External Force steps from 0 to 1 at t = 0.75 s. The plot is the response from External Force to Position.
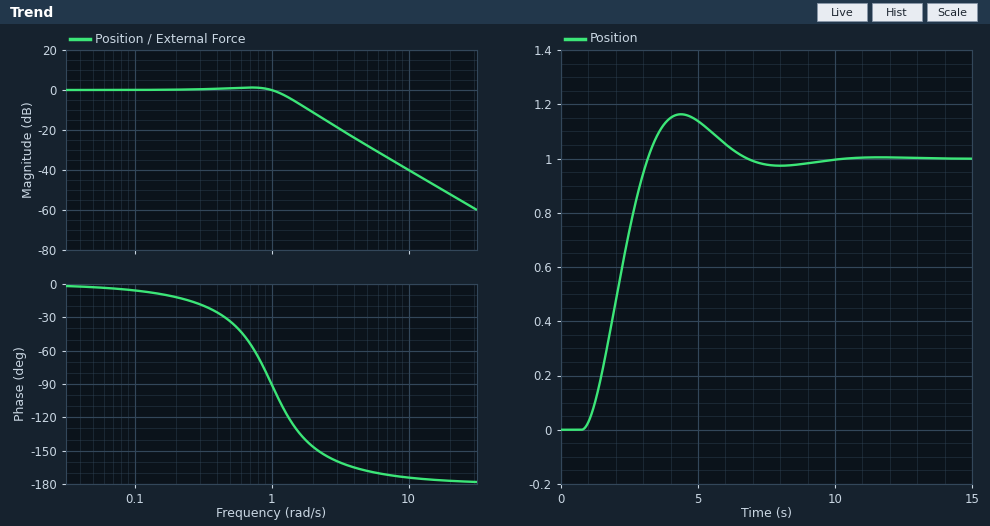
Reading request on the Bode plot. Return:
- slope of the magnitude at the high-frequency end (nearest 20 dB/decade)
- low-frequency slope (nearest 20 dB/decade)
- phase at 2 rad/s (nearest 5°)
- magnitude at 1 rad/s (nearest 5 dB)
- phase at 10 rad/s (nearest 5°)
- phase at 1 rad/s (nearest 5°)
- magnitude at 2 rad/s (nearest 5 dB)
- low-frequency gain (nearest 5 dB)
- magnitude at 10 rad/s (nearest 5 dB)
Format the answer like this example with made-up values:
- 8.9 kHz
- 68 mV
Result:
- -40 dB/decade
- 0 dB/decade
- -145°
- 0 dB
- -175°
- -90°
- -10 dB
- 0 dB
- -40 dB
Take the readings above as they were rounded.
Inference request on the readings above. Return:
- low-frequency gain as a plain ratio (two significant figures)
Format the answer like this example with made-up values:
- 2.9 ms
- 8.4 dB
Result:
- 1.0
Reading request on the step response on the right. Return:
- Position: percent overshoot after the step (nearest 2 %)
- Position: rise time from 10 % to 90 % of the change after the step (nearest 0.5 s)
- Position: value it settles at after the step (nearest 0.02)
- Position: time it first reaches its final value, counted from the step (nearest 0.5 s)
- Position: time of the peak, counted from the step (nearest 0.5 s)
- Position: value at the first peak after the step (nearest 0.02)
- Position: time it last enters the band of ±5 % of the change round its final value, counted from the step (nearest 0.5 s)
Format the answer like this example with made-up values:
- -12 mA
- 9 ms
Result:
- 16 %
- 1.5 s
- 1.00
- 2.5 s
- 3.5 s
- 1.16
- 5.5 s
